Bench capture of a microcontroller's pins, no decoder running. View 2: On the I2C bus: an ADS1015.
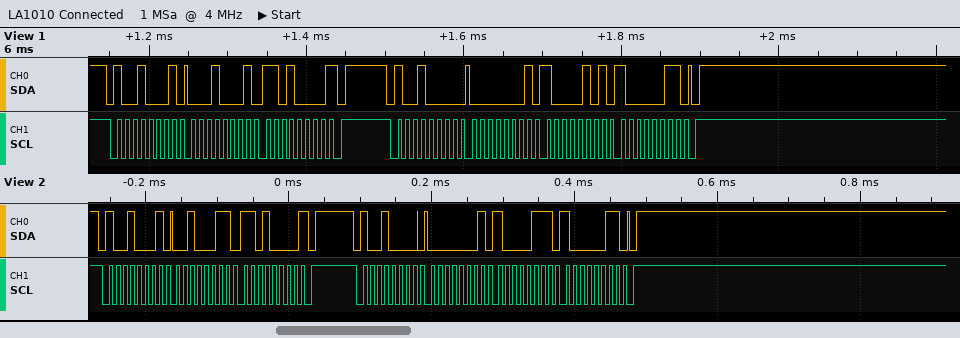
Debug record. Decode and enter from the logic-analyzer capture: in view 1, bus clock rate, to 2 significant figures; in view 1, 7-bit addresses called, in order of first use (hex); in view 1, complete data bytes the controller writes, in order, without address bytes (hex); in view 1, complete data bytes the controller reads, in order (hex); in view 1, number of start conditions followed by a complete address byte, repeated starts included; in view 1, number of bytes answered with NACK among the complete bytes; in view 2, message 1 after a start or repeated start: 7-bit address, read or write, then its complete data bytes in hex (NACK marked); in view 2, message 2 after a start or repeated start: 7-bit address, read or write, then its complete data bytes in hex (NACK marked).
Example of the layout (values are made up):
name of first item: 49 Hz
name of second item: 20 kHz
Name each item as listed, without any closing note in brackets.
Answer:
in view 1, bus clock rate, to 2 significant figures: 100 kHz
in view 1, 7-bit addresses called, in order of first use: 0x48
in view 1, complete data bytes the controller writes, in order, without address bytes: 01 85 83
in view 1, complete data bytes the controller reads, in order: 11 D0
in view 1, number of start conditions followed by a complete address byte, repeated starts included: 2
in view 1, number of bytes answered with NACK among the complete bytes: 1
in view 2, message 1 after a start or repeated start: 7-bit address, read or write, then its complete data bytes in hex: 0x48 read: 23 D0 NACK
in view 2, message 2 after a start or repeated start: 7-bit address, read or write, then its complete data bytes in hex: 0x48 write: 01 87 83
